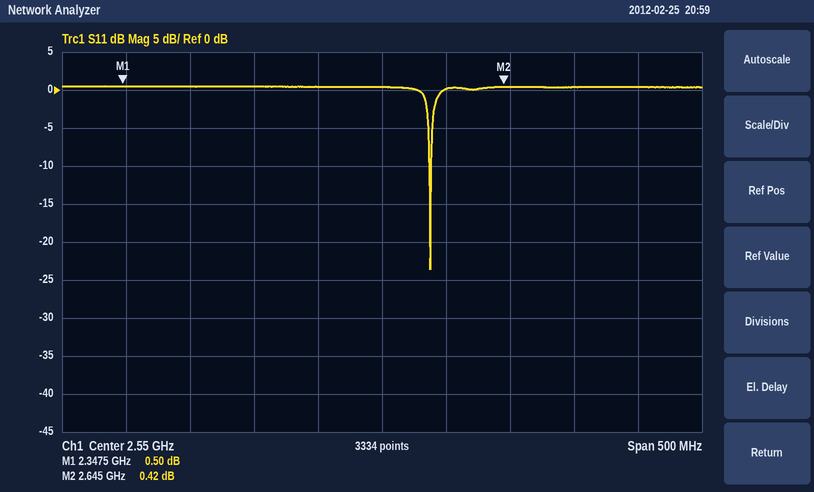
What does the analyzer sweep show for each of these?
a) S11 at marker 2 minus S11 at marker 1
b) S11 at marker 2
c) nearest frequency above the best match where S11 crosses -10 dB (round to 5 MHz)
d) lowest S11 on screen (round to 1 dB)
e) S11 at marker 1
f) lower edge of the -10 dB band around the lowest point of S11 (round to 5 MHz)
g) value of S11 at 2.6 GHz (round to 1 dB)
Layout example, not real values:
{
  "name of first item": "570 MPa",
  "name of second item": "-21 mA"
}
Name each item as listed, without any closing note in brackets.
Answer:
{
  "S11 at marker 2 minus S11 at marker 1": "-0.08 dB",
  "S11 at marker 2": "0.42 dB",
  "nearest frequency above the best match where S11 crosses -10 dB": "2.590 GHz",
  "lowest S11 on screen": "-24 dB",
  "S11 at marker 1": "0.50 dB",
  "lower edge of the -10 dB band around the lowest point of S11": "2.585 GHz",
  "value of S11 at 2.6 GHz": "0 dB"
}
